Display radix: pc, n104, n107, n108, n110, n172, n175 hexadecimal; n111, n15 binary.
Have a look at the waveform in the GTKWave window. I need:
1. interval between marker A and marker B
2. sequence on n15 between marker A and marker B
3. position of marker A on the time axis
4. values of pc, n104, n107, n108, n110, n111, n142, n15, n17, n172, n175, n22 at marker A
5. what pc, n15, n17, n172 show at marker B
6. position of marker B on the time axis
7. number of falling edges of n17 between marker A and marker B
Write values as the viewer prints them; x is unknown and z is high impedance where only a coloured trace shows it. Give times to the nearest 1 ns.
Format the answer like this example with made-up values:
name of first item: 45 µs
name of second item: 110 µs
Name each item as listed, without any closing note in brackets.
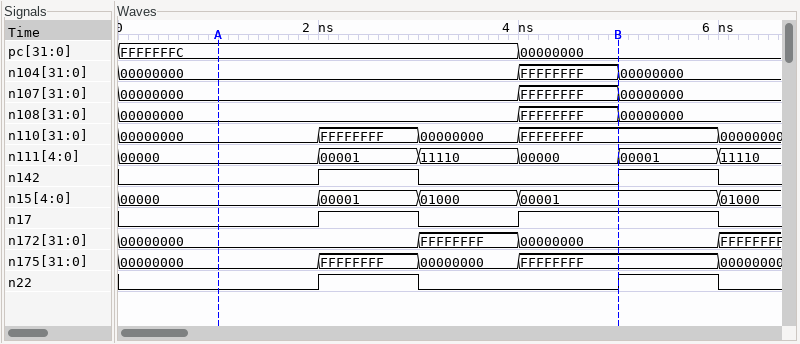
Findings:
interval between marker A and marker B: 4 ns
sequence on n15 between marker A and marker B: 00000, 00001, 01000, 00001
position of marker A on the time axis: 1 ns
values of pc, n104, n107, n108, n110, n111, n142, n15, n17, n172, n175, n22 at marker A: pc=FFFFFFFC, n104=00000000, n107=00000000, n108=00000000, n110=00000000, n111=00000, n142=0, n15=00000, n17=0, n172=00000000, n175=00000000, n22=0
what pc, n15, n17, n172 show at marker B: pc=00000000, n15=00001, n17=1, n172=00000000
position of marker B on the time axis: 5 ns
number of falling edges of n17 between marker A and marker B: 1
